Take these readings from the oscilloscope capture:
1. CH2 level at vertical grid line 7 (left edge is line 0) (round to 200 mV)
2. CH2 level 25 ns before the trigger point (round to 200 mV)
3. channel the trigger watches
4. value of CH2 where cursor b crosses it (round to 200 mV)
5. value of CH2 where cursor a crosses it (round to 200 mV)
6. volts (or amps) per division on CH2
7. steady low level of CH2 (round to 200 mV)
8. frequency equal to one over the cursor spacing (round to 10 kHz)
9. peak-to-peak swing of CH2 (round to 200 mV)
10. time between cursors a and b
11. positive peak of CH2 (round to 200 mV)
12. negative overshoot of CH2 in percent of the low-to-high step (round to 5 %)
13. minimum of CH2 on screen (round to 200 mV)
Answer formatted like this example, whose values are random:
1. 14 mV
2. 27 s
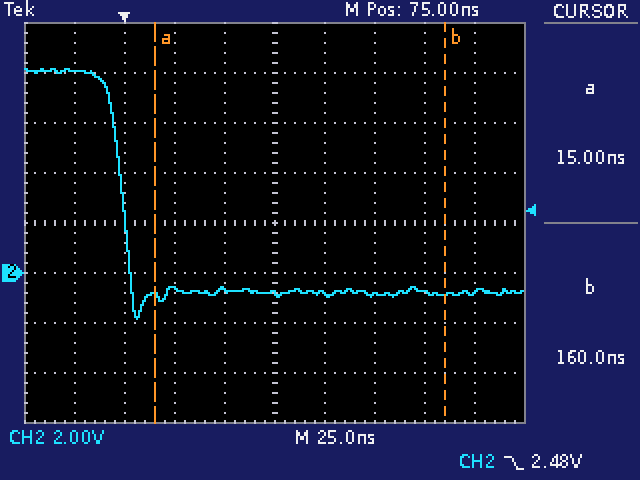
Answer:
1. -800 mV
2. 8.0 V
3. CH2
4. -800 mV
5. -1.0 V
6. 2 V
7. -800 mV
8. 6.90 MHz
9. 10.0 V
10. 145.0 ns
11. 8.2 V
12. 10 %
13. -1.8 V
